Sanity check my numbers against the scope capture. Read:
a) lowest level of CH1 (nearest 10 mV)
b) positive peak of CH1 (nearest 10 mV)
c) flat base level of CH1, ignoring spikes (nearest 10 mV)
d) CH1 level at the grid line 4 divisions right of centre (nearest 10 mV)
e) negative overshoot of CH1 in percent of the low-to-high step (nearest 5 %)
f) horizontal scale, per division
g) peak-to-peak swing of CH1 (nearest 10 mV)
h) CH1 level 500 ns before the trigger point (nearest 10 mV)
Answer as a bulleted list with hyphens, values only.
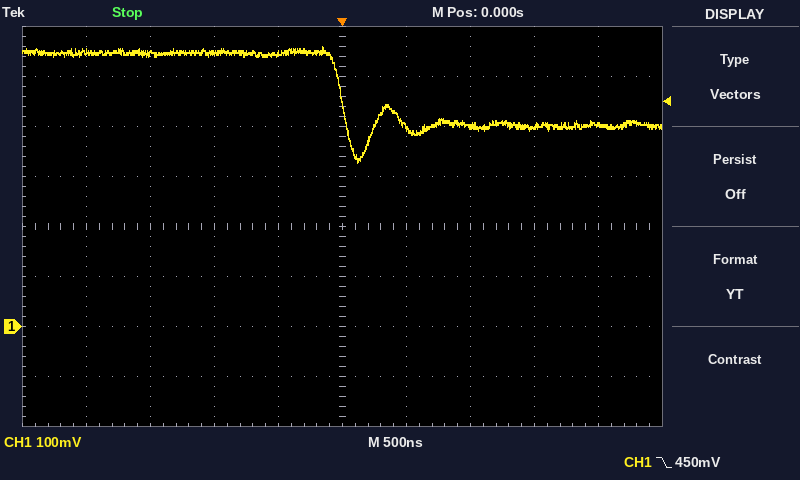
- 330 mV
- 560 mV
- 400 mV
- 400 mV
- 50 %
- 500 ns
- 230 mV
- 550 mV
